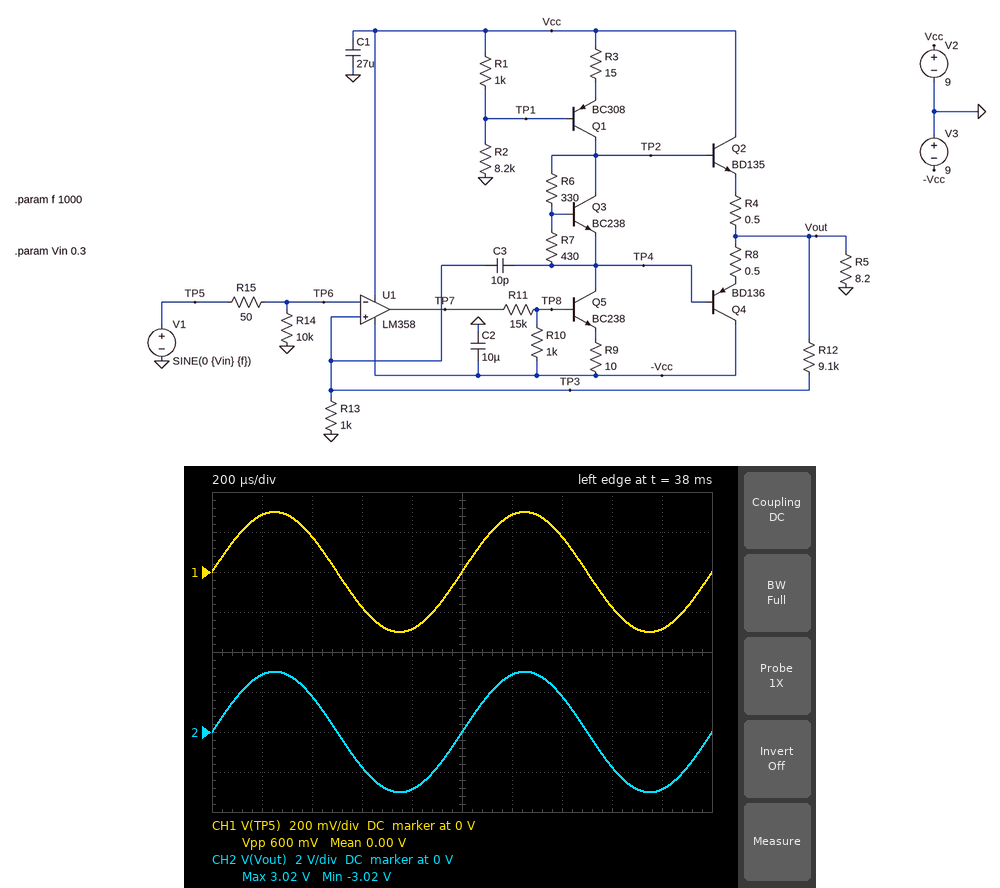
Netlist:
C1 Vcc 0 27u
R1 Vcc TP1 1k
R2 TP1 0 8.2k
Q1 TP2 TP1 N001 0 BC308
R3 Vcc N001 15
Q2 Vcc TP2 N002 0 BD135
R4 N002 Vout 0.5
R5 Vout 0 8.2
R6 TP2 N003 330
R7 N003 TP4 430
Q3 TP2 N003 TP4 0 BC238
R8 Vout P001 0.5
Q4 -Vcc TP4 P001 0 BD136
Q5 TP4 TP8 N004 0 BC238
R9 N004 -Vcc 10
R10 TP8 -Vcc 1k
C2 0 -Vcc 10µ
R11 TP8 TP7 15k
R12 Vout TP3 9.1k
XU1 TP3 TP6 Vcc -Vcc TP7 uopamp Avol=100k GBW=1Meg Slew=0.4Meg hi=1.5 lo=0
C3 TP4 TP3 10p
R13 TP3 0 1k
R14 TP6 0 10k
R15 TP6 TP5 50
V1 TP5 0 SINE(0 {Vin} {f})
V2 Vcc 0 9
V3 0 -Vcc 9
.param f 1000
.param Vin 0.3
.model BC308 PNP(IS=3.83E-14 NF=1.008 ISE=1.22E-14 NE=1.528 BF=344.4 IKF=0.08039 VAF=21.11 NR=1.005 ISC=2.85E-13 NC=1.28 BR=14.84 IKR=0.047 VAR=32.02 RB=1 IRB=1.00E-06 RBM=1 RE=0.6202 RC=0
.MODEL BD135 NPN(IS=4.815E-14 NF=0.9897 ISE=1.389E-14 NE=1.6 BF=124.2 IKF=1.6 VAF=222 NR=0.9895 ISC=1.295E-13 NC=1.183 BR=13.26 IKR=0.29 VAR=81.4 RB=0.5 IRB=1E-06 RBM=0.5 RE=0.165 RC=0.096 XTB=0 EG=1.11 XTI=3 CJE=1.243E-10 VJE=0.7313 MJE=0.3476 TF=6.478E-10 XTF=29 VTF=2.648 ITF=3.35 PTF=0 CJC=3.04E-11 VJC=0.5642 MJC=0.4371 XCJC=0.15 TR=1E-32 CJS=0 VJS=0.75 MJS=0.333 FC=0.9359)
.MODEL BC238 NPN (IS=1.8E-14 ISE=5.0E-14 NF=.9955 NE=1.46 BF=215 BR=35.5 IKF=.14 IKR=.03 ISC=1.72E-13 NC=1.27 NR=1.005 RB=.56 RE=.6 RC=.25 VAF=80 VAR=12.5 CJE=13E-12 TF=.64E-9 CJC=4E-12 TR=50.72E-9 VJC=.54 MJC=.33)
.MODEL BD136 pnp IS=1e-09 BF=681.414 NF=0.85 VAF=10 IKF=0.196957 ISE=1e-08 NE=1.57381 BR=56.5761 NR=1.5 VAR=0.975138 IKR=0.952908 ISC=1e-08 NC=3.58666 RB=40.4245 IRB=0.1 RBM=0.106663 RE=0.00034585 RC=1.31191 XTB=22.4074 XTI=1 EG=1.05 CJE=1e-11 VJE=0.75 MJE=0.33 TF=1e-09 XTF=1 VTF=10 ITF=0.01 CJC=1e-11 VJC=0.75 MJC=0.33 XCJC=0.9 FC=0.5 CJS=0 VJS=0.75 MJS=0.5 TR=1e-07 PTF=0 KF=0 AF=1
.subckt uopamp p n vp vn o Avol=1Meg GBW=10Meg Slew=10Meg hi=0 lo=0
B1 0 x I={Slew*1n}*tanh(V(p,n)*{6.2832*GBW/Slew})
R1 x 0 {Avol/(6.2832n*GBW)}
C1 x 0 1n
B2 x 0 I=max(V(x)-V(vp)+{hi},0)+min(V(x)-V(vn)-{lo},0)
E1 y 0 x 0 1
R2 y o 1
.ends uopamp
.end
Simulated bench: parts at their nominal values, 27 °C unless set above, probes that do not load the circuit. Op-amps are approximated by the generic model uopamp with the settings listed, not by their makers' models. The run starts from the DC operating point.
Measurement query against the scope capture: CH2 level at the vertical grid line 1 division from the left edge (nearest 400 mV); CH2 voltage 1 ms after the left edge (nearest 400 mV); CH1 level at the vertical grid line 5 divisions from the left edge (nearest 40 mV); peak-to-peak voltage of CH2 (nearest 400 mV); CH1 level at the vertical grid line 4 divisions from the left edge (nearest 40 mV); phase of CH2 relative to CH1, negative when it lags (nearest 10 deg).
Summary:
2.8 V
0 V
0 V
6.0 V
-280 mV
0 deg
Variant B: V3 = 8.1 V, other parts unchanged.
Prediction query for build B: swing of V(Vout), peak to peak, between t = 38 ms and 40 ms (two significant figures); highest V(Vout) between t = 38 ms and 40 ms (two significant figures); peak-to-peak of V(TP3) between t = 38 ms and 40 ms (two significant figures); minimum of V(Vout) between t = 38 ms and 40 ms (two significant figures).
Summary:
4.3 V
3.0 V
420 mV
-1.3 V
